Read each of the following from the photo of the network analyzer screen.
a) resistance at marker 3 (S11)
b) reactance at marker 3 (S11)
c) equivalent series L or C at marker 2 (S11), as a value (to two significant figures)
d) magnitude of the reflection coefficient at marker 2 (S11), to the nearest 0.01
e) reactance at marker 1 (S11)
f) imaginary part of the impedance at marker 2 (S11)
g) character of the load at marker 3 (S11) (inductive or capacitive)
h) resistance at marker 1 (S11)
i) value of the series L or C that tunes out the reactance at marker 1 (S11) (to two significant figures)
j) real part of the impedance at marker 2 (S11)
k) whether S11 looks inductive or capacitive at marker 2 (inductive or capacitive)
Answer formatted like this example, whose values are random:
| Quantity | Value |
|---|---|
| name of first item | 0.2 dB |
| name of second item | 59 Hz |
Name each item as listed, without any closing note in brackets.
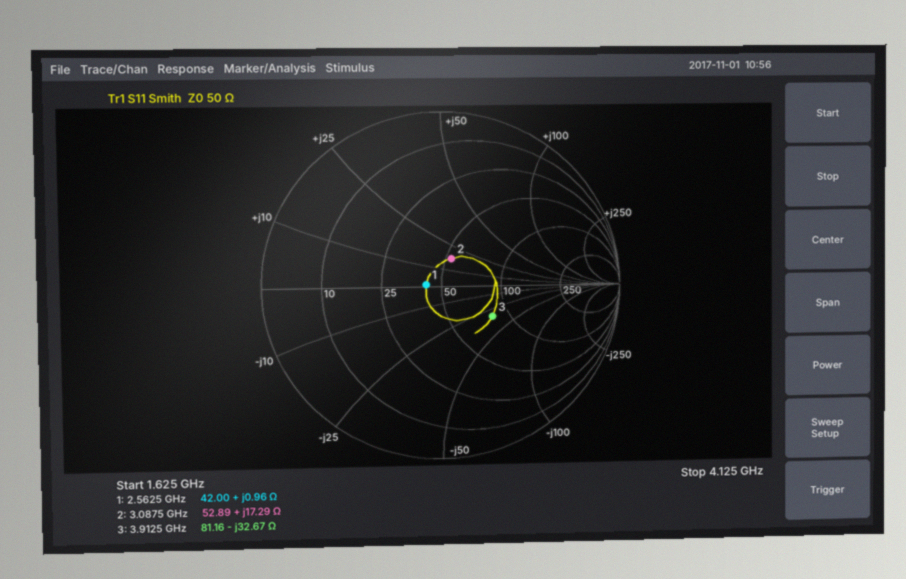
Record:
| Quantity | Value |
|---|---|
| resistance at marker 3 | 81.16 Ω |
| reactance at marker 3 | -32.67 Ω |
| equivalent series L or C at marker 2 (S11), as a value | 890 pH |
| magnitude of the reflection coefficient at marker 2 (S11), to the nearest 0.01 | 0.17 |
| reactance at marker 1 | +0.96 Ω |
| imaginary part of the impedance at marker 2 | +17.29 Ω |
| character of the load at marker 3 (S11) | capacitive |
| resistance at marker 1 | 42.00 Ω |
| value of the series L or C that tunes out the reactance at marker 1 (S11) | 65 pF |
| real part of the impedance at marker 2 | 52.89 Ω |
| whether S11 looks inductive or capacitive at marker 2 | inductive |
